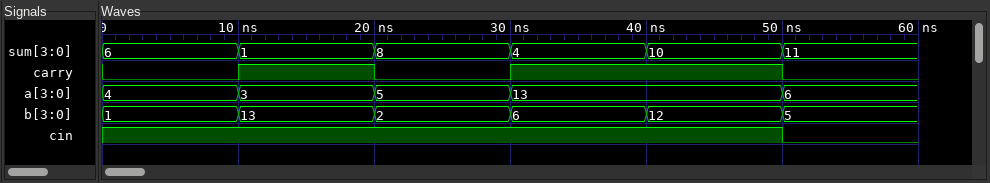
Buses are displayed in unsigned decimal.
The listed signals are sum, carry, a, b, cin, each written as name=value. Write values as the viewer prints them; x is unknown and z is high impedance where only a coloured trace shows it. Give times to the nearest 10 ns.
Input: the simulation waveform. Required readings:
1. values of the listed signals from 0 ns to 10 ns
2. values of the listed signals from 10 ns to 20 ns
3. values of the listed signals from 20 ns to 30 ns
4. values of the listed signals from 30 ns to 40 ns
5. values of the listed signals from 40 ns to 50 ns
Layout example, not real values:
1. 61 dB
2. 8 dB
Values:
1. sum=6, carry=0, a=4, b=1, cin=1
2. sum=1, carry=1, a=3, b=13, cin=1
3. sum=8, carry=0, a=5, b=2, cin=1
4. sum=4, carry=1, a=13, b=6, cin=1
5. sum=10, carry=1, a=13, b=12, cin=1
